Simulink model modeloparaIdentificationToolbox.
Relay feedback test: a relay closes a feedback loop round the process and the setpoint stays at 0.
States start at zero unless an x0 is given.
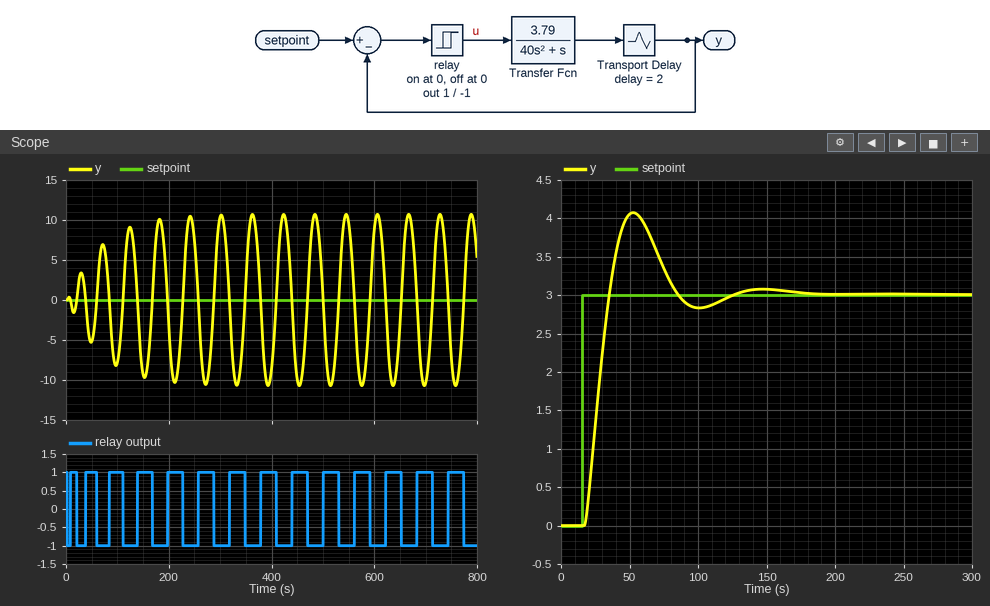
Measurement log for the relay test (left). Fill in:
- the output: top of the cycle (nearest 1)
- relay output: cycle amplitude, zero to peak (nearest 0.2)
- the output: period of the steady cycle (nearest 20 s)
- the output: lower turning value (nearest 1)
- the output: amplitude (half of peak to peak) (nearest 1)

11
1.0
60 s
-11
11
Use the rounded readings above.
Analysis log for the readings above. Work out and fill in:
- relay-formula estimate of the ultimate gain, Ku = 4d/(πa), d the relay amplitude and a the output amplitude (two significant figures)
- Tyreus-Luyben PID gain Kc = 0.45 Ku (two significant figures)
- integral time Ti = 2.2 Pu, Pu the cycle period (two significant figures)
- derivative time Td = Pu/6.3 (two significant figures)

0.12
0.054
130 s
9.5 s
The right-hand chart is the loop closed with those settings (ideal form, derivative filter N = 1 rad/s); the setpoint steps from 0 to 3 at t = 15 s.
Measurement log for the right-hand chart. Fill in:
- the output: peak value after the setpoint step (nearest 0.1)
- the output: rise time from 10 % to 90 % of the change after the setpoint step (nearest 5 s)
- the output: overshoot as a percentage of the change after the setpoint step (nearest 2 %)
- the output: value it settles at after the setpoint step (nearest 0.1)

4.1
15 s
36 %
3.0
